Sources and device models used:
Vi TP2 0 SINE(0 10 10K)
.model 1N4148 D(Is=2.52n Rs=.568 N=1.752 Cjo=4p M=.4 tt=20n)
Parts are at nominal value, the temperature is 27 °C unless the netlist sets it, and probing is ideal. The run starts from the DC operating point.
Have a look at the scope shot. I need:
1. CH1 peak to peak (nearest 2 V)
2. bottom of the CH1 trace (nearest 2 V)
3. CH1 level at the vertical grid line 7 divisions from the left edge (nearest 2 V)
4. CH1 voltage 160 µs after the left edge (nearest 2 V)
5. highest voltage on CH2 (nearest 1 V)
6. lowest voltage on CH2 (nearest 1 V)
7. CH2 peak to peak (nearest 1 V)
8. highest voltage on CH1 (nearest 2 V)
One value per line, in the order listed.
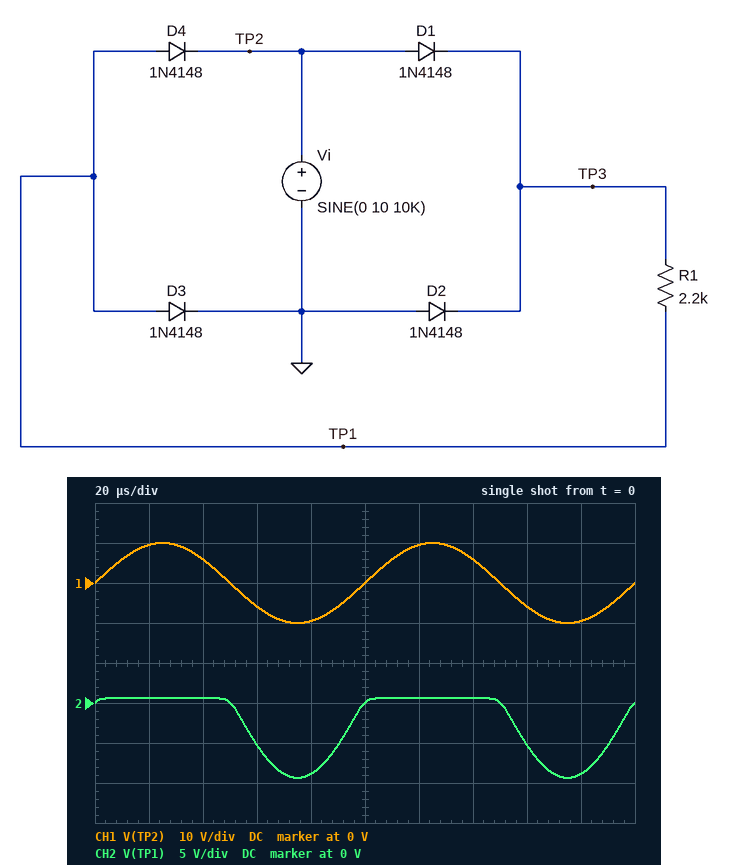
20 V
-10 V
6 V
-6 V
1 V
-9 V
10 V
10 V
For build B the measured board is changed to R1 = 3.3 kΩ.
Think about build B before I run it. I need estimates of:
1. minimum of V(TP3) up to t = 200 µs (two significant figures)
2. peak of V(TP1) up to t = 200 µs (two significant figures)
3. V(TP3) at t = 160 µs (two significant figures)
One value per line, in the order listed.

-630 mV
630 mV
-600 mV
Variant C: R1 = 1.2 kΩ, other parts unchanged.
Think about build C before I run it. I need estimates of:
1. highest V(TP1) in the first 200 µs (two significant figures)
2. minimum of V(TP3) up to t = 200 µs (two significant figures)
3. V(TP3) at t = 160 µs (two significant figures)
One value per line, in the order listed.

680 mV
-680 mV
-650 mV
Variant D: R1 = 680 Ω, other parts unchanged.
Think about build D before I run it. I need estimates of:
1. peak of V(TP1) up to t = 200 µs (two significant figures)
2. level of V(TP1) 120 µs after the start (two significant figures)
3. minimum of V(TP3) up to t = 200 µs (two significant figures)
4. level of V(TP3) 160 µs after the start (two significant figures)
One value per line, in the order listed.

710 mV
700 mV
-710 mV
-670 mV
